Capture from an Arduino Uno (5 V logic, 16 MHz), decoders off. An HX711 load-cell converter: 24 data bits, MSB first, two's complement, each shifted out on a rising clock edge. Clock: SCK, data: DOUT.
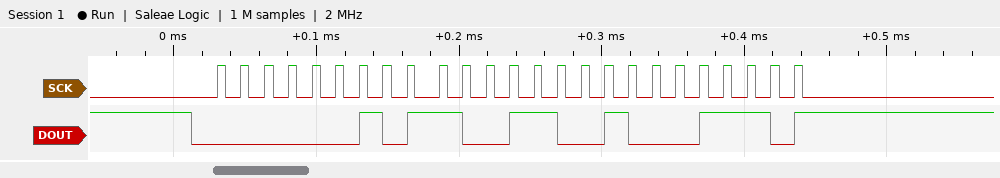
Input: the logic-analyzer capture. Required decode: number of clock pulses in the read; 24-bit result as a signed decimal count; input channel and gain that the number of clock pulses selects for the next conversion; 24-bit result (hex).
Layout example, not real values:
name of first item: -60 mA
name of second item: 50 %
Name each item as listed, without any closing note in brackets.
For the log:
number of clock pulses in the read: 25
24-bit result as a signed decimal count: 183438
input channel and gain that the number of clock pulses selects for the next conversion: channel A, gain 128
24-bit result: 0x02CC8E
